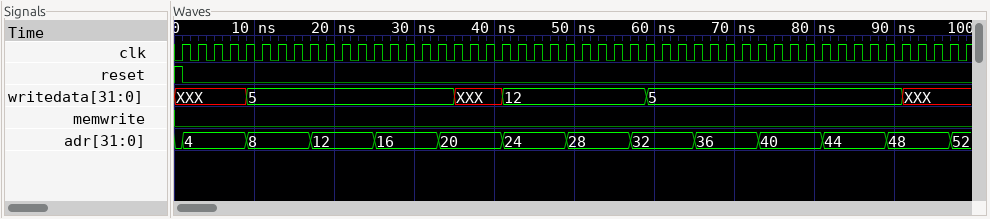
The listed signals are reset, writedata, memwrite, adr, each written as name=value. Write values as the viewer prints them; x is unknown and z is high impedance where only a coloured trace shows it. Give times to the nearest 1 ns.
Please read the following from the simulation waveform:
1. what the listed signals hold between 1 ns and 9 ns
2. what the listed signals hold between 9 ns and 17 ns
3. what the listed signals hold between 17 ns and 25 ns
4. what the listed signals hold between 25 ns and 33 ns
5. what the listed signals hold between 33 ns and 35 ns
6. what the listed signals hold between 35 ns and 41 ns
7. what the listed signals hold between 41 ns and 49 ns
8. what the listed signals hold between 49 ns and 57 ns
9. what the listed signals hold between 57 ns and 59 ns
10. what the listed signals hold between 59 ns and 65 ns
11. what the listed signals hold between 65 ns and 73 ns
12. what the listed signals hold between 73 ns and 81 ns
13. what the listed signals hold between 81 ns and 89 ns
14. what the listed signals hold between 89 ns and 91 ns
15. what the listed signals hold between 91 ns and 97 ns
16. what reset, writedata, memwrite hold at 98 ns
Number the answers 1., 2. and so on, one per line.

1. reset=0, writedata=XXX, memwrite=0, adr=4
2. reset=0, writedata=5, memwrite=0, adr=8
3. reset=0, writedata=5, memwrite=0, adr=12
4. reset=0, writedata=5, memwrite=0, adr=16
5. reset=0, writedata=5, memwrite=0, adr=20
6. reset=0, writedata=XXX, memwrite=0, adr=20
7. reset=0, writedata=12, memwrite=0, adr=24
8. reset=0, writedata=12, memwrite=0, adr=28
9. reset=0, writedata=12, memwrite=0, adr=32
10. reset=0, writedata=5, memwrite=0, adr=32
11. reset=0, writedata=5, memwrite=0, adr=36
12. reset=0, writedata=5, memwrite=0, adr=40
13. reset=0, writedata=5, memwrite=0, adr=44
14. reset=0, writedata=5, memwrite=0, adr=48
15. reset=0, writedata=XXX, memwrite=0, adr=48
16. reset=0, writedata=XXX, memwrite=0
